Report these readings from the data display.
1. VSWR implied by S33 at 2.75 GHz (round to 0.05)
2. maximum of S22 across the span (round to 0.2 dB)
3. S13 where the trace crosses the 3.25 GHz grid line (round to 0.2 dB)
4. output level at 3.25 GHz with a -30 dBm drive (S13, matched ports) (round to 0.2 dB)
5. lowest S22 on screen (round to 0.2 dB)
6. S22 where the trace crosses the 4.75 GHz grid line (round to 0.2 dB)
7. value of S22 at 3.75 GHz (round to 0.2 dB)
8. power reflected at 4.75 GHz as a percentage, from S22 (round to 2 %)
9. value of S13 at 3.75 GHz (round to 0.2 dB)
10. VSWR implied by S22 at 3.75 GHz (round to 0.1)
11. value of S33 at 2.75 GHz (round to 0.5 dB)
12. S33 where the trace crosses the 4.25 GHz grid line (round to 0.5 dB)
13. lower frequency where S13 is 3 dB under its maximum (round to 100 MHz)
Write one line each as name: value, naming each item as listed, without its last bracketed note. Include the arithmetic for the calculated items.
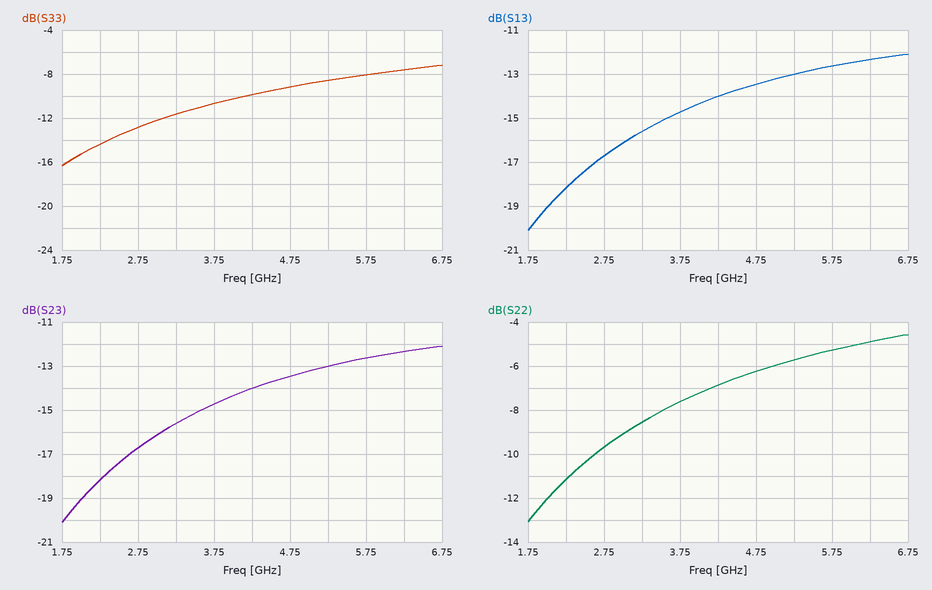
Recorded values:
VSWR implied by S33 at 2.75 GHz: |Γ| = 10^(-13/20) = 0.2239; VSWR = (1 + 0.2239)/(1 − 0.2239) ≈ 1.58, so 1.60 to the nearest 0.05
maximum of S22 across the span: -4.6 dB
S13 where the trace crosses the 3.25 GHz grid line: -15.6 dB
output level at 3.25 GHz with a -30 dBm drive (S13, matched ports): -30 dBm + (-15.6 dB) = -45.6 dBm
lowest S22 on screen: -13.0 dB
S22 where the trace crosses the 4.75 GHz grid line: -6.2 dB
value of S22 at 3.75 GHz: -7.6 dB
power reflected at 4.75 GHz as a percentage, from S22: 10^(-6.2/10) ≈ 24 %
value of S13 at 3.75 GHz: -14.8 dB
VSWR implied by S22 at 3.75 GHz: |Γ| = 10^(-7.6/20) = 0.4169; VSWR = (1 + 0.4169)/(1 − 0.4169) ≈ 2.4
value of S33 at 2.75 GHz: -13.0 dB
S33 where the trace crosses the 4.25 GHz grid line: -10.0 dB
lower frequency where S13 is 3 dB under its maximum: 3.5 GHz
